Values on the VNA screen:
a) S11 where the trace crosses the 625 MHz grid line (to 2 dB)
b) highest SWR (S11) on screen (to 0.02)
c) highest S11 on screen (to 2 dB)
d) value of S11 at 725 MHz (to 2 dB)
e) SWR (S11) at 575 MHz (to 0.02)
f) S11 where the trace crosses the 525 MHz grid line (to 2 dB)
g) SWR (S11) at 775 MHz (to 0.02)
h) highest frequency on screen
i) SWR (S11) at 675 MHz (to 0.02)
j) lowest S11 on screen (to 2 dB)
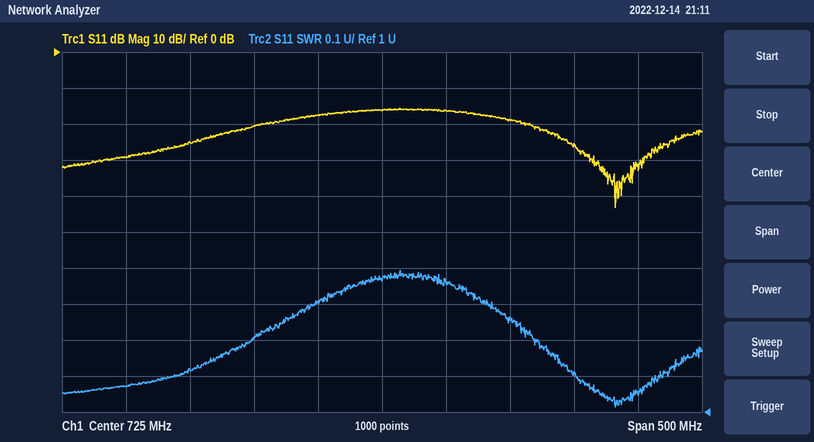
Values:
-20 dB
1.40
-16 dB
-16 dB
1.12
-30 dB
1.36
975 MHz
1.30
-44 dB
